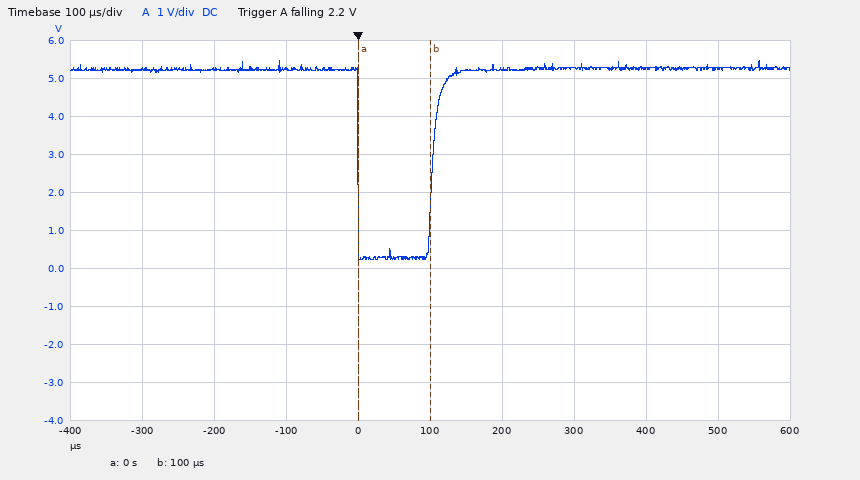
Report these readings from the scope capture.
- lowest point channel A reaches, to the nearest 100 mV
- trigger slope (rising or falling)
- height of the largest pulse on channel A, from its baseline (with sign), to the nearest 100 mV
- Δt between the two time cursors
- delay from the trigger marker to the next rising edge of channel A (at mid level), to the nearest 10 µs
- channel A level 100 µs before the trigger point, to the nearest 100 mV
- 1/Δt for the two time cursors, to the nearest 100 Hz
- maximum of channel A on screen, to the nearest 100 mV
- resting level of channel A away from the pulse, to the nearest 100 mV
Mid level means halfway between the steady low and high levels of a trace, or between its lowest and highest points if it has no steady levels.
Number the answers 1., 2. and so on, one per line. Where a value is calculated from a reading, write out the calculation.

1. 200 mV
2. falling
3. 200 mV − (5.2 V) = -5.0 V
4. 100 µs − (0 s) = 100 µs
5. 100 µs
6. 5.2 V
7. 1 / 100 µs ≈ 10.0 kHz
8. 5.5 V
9. 5.2 V
